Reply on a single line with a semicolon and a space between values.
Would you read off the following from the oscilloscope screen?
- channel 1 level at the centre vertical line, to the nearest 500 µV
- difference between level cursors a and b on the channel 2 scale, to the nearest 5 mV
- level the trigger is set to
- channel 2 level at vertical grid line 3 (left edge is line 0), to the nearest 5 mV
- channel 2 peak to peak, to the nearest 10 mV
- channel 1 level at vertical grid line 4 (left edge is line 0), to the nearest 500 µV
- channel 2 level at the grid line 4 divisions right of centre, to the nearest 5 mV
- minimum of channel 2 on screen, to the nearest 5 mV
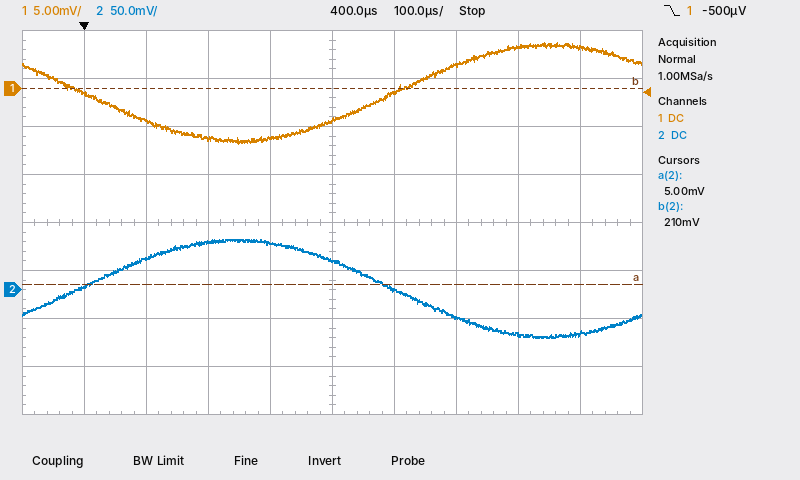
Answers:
-3.5 mV; 205 mV; -500 µV; 50 mV; 100 mV; -5.0 mV; -45 mV; -50 mV
